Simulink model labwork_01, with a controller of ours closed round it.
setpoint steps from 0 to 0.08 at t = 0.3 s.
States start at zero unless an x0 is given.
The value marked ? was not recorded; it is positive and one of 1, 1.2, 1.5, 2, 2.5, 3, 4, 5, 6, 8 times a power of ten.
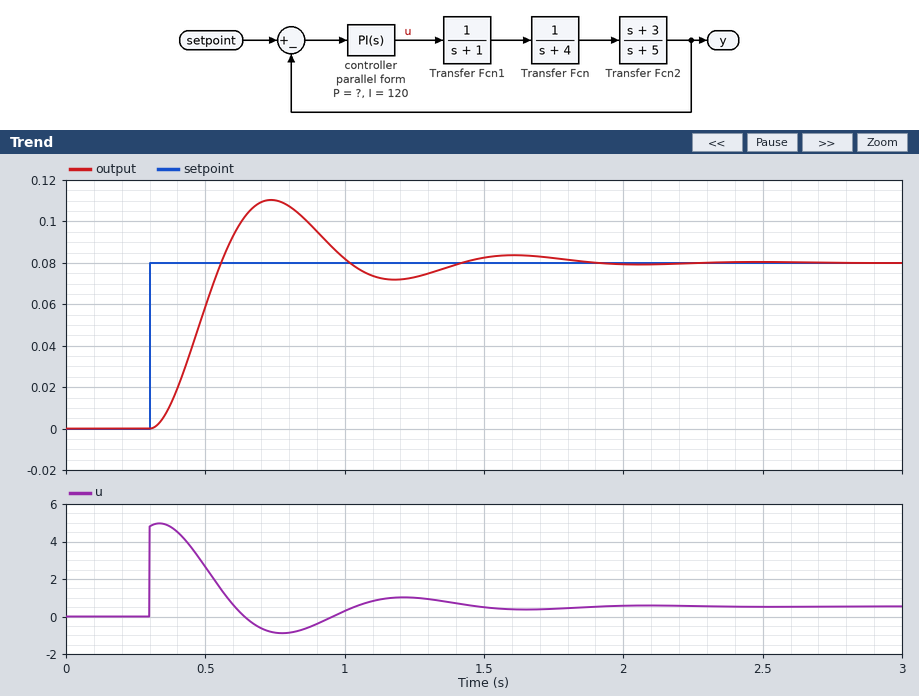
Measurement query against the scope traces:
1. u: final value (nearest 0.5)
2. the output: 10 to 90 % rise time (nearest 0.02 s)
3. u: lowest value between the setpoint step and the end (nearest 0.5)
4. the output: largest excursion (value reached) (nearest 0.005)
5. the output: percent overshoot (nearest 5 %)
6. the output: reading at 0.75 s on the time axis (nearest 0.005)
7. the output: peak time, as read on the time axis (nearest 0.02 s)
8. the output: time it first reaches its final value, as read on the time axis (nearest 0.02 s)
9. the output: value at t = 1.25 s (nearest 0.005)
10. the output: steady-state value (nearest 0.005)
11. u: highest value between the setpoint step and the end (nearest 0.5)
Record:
0.5
0.18 s
-1.0
0.110
40 %
0.110
0.74 s
0.56 s
0.075
0.080
5.0
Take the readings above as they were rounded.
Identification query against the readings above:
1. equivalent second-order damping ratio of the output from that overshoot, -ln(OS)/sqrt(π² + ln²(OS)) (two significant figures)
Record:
0.28
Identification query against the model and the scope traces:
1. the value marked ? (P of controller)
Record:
60
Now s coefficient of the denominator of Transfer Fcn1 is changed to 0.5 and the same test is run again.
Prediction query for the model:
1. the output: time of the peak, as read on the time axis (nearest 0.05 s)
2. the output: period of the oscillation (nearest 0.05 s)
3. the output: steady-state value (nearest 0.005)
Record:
0.60 s
0.60 s
0.080
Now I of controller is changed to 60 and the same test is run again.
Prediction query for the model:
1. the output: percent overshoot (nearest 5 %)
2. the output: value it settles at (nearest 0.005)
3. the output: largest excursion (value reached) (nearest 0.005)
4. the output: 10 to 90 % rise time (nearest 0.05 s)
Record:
25 %
0.080
0.100
0.20 s
